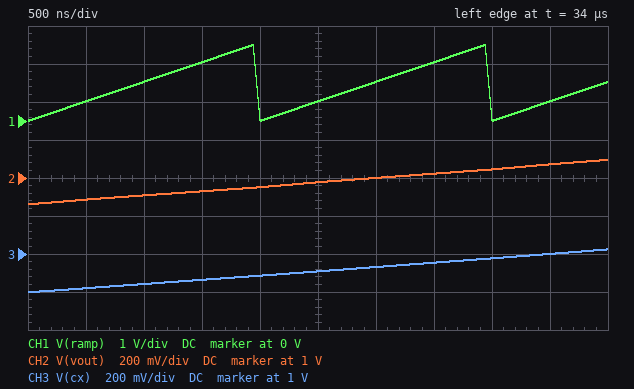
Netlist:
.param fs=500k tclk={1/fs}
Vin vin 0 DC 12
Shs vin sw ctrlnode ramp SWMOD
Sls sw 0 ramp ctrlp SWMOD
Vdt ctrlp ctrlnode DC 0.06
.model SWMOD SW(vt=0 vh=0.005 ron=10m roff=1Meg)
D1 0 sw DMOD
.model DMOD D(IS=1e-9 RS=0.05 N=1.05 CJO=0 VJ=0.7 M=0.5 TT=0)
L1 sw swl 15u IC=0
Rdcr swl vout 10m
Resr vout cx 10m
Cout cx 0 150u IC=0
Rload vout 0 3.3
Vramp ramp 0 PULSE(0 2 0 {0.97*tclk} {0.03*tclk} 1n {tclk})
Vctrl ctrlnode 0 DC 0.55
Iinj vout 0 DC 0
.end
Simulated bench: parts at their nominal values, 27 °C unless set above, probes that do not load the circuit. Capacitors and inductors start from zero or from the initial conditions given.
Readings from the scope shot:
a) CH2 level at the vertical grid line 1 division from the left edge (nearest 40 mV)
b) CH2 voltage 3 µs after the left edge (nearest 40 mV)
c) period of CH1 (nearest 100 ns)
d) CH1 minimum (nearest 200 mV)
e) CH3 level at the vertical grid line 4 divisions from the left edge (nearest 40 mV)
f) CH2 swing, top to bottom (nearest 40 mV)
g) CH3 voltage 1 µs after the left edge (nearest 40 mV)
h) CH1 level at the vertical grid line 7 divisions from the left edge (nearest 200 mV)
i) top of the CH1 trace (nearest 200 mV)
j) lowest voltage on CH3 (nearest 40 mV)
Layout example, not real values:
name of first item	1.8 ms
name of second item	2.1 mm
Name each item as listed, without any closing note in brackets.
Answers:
CH2 level at the vertical grid line 1 division from the left edge	880 mV
CH2 voltage 3 µs after the left edge	1.00 V
period of CH1	2.0 µs
CH1 minimum	0 V
CH3 level at the vertical grid line 4 divisions from the left edge	880 mV
CH2 swing, top to bottom	240 mV
CH3 voltage 1 µs after the left edge	840 mV
CH1 level at the vertical grid line 7 divisions from the left edge	1.6 V
top of the CH1 trace	2.0 V
lowest voltage on CH3	800 mV
